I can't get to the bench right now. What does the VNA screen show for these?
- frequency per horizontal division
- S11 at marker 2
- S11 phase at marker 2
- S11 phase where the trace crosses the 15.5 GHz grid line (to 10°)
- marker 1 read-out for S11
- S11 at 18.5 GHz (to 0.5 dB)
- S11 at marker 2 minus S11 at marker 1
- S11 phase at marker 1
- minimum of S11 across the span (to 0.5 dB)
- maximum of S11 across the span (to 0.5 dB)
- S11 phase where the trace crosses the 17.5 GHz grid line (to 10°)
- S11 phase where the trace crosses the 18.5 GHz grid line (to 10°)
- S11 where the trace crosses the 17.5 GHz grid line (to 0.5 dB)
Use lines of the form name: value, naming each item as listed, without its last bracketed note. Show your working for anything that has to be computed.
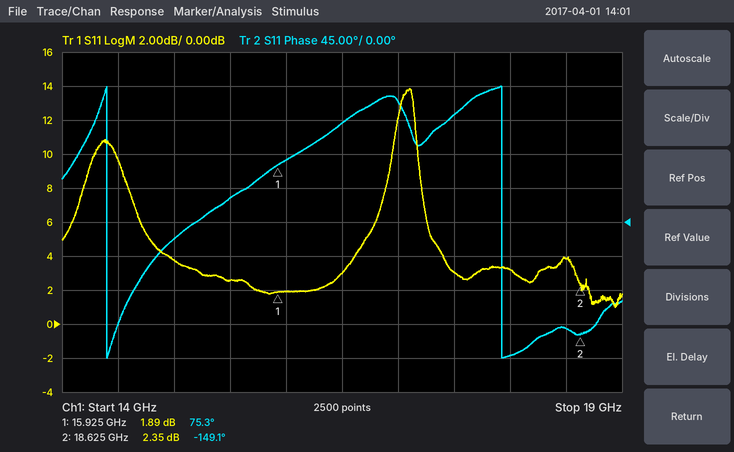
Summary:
frequency per horizontal division: 500 MHz
S11 at marker 2: 2.35 dB
S11 phase at marker 2: -149.1°
S11 phase where the trace crosses the 15.5 GHz grid line: 30°
marker 1 read-out for S11: 1.89 dB
S11 at 18.5 GHz: 4.0 dB
S11 at marker 2 minus S11 at marker 1: 2.35 − (1.89) = 0.46 dB
S11 phase at marker 1: 75.3°
minimum of S11 across the span: 1.0 dB
maximum of S11 across the span: 14.0 dB
S11 phase where the trace crosses the 17.5 GHz grid line: 140°
S11 phase where the trace crosses the 18.5 GHz grid line: -140°
S11 where the trace crosses the 17.5 GHz grid line: 3.0 dB
